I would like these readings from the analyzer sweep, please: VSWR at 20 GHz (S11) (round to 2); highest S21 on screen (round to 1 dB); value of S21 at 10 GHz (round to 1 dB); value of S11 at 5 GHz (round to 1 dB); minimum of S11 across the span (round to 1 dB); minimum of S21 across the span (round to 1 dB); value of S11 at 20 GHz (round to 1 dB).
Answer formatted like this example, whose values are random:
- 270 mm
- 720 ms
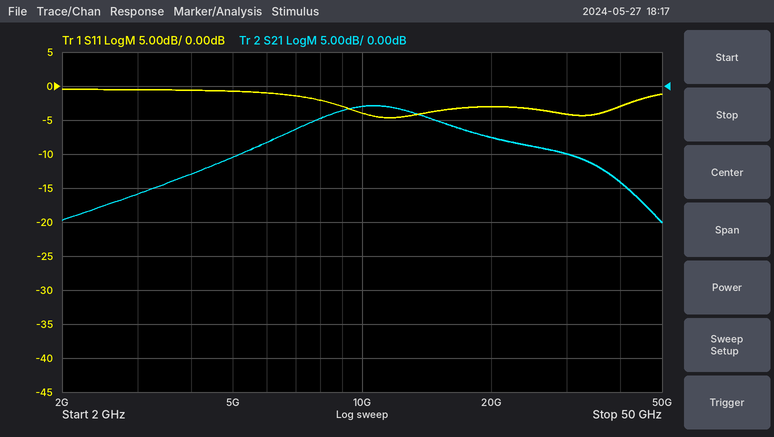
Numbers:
- 6
- -3 dB
- -3 dB
- -1 dB
- -5 dB
- -20 dB
- -3 dB
